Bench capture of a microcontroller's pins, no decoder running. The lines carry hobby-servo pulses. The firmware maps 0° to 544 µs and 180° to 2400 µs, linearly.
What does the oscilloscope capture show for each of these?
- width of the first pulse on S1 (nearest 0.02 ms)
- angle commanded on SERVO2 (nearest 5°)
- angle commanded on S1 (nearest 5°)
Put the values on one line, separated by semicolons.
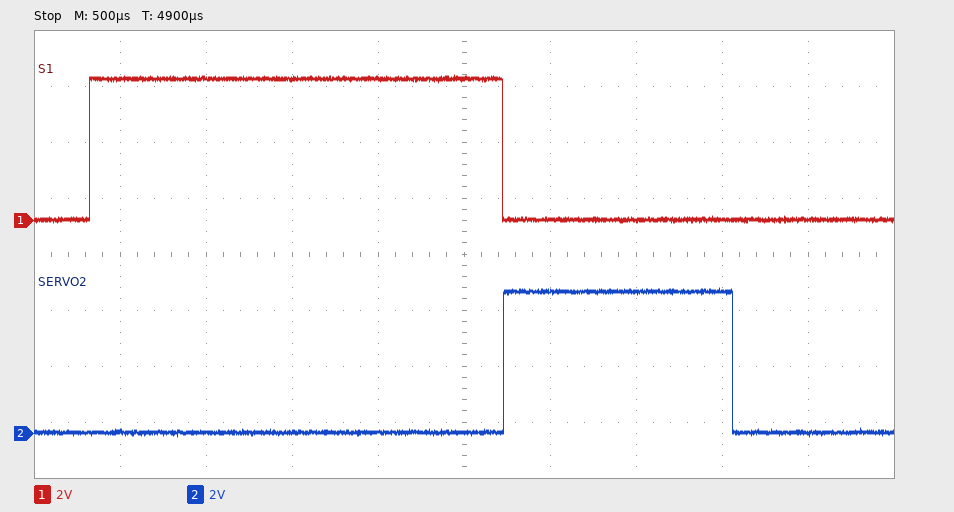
2.40 ms; 75°; 180°
